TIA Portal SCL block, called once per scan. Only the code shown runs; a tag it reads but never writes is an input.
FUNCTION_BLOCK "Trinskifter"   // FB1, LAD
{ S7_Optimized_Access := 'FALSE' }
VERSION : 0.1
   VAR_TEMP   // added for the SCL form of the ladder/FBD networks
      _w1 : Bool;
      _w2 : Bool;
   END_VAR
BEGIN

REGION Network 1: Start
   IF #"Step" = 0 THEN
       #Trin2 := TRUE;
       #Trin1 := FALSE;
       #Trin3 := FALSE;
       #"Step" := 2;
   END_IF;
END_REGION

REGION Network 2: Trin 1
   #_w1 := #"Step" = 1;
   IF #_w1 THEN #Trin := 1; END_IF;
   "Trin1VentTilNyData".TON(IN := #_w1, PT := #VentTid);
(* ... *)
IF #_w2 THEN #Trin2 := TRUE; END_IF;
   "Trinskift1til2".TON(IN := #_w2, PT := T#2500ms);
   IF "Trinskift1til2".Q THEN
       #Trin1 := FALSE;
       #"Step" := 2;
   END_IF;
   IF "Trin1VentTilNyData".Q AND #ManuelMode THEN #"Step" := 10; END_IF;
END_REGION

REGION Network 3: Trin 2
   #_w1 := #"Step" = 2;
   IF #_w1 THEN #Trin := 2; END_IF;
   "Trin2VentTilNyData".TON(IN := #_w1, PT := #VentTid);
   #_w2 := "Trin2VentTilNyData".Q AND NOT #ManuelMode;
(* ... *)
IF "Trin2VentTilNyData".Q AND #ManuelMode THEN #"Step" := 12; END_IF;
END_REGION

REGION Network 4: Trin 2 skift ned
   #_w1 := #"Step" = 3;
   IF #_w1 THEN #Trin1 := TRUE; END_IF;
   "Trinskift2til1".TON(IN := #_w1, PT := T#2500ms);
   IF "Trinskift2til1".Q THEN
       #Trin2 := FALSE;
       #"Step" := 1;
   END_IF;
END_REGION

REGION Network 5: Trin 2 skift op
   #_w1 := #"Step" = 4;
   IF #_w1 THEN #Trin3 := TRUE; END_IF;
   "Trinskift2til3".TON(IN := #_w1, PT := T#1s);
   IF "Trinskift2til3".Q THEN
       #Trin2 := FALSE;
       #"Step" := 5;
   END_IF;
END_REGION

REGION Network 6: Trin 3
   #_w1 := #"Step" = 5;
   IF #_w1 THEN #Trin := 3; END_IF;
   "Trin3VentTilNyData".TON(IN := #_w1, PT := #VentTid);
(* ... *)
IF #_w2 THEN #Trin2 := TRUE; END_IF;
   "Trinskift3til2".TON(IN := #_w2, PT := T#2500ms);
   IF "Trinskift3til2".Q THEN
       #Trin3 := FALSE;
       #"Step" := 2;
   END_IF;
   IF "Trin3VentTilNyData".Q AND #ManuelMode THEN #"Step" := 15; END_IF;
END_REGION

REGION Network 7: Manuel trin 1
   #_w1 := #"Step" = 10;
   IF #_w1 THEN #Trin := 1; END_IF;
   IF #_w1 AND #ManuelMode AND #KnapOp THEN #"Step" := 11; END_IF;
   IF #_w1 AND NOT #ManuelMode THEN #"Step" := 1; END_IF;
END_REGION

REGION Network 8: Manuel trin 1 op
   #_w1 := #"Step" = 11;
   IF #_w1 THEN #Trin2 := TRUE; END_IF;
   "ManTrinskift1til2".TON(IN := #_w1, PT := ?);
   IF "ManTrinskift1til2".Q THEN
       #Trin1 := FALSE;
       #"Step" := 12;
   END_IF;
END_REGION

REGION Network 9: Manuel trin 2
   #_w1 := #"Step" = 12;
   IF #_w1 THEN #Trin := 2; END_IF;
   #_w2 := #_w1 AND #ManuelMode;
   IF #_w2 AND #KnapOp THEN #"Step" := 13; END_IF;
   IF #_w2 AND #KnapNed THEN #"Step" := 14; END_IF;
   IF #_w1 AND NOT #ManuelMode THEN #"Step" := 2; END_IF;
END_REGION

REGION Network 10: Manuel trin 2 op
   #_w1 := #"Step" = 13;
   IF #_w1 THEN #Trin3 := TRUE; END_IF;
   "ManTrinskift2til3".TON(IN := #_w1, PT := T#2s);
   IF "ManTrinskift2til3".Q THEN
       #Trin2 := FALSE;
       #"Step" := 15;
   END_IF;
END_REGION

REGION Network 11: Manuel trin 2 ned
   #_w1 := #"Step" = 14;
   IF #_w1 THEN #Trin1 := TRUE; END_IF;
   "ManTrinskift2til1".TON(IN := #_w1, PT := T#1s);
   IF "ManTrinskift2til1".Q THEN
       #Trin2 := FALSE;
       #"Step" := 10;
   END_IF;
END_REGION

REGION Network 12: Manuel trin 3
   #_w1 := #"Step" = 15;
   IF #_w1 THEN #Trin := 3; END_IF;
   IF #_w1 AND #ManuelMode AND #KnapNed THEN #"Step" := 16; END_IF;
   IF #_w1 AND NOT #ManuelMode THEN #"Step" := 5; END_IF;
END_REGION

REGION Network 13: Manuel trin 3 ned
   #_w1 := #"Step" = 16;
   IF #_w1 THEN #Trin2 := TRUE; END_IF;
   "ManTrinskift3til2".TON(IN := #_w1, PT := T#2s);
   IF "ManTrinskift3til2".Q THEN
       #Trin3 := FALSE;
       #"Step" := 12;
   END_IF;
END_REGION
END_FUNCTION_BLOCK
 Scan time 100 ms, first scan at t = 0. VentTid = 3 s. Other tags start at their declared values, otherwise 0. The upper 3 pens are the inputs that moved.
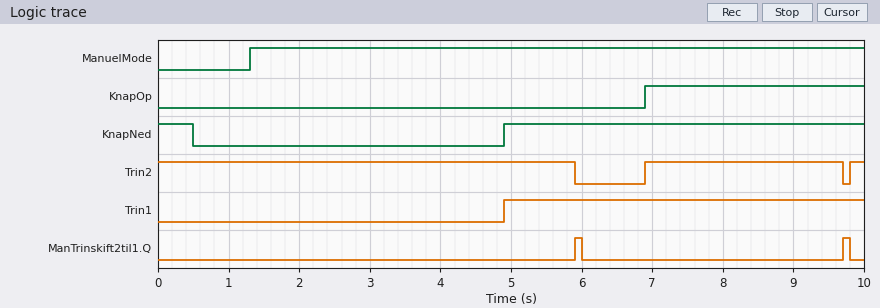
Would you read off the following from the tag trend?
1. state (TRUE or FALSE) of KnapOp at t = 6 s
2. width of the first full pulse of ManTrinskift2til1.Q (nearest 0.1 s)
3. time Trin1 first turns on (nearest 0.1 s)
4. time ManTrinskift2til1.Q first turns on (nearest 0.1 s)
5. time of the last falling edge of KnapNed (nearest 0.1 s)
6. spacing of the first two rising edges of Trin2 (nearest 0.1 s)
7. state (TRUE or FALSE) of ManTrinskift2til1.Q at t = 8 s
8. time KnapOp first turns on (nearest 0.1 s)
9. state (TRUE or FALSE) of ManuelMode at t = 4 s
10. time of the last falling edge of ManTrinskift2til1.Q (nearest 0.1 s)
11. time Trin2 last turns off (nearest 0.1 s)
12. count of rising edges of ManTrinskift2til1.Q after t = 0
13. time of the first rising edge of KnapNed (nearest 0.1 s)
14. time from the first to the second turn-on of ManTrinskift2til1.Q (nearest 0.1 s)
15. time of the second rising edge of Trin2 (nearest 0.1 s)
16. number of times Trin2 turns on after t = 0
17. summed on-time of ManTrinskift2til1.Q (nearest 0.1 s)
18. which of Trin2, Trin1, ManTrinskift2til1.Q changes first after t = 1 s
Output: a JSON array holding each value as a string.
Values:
["FALSE", "0.1 s", "4.9 s", "5.9 s", "0.5 s", "2.9 s", "FALSE", "6.9 s", "TRUE", "9.8 s", "9.7 s", "2", "4.9 s", "3.8 s", "9.8 s", "2", "0.2 s", "Trin1"]
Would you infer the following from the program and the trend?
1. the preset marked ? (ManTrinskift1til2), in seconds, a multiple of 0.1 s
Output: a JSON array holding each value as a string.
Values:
["1.8 s"]
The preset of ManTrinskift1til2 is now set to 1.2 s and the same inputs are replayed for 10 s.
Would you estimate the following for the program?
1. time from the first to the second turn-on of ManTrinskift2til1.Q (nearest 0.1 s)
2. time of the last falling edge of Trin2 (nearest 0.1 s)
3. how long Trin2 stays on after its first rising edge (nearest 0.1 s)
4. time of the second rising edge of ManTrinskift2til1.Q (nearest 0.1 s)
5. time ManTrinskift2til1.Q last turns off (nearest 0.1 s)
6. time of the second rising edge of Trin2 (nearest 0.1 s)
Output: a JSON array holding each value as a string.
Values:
["3.2 s", "9.1 s", "2.2 s", "9.1 s", "9.2 s", "9.2 s"]
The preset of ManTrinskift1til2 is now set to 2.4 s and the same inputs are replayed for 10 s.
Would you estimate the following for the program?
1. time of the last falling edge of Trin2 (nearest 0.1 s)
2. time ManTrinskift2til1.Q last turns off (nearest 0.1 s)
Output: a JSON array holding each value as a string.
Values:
["5.9 s", "6.0 s"]
